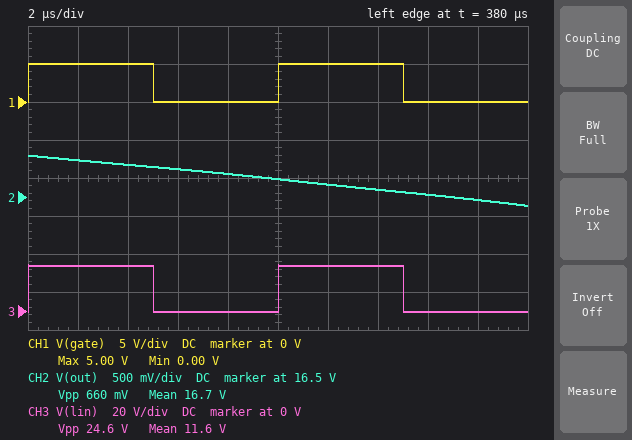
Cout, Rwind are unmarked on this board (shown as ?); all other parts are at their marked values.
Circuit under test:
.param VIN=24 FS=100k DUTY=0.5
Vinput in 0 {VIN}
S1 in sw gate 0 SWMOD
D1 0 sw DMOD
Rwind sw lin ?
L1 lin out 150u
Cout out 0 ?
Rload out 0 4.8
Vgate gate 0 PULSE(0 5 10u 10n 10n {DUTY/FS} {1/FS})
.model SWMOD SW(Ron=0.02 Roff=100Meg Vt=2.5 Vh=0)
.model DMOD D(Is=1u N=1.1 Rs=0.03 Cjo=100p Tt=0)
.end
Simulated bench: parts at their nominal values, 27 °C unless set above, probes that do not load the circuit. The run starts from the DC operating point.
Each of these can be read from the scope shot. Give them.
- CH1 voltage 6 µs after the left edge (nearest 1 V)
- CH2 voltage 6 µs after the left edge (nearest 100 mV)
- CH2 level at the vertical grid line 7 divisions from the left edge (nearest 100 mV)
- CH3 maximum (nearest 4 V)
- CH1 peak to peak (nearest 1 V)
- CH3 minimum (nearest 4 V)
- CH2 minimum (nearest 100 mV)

0 V
16.9 V
16.6 V
24 V
5 V
0 V
16.4 V
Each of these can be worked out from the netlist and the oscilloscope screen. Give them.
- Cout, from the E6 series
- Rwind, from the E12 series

68 µF
0.082 Ω
